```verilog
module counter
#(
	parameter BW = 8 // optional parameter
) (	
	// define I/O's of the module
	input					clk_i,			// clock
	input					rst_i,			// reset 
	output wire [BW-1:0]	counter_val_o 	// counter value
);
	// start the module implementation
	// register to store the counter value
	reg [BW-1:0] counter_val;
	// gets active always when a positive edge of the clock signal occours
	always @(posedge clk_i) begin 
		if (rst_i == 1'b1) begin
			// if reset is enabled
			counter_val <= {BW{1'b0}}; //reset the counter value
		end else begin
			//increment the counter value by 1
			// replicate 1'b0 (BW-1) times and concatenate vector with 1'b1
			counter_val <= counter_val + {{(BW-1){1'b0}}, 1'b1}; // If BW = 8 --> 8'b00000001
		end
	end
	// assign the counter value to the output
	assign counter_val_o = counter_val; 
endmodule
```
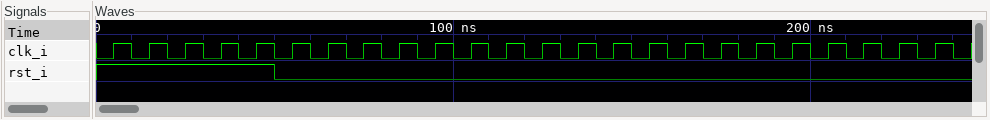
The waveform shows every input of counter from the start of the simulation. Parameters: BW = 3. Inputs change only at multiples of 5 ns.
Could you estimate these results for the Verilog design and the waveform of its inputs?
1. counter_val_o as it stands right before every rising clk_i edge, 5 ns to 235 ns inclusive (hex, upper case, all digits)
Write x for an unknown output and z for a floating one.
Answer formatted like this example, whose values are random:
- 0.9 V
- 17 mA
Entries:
- x, 0, 0, 0, 0, 0, 1, 2, 3, 4, 5, 6, 7, 0, 1, 2, 3, 4, 5, 6, 7, 0, 1, 2
